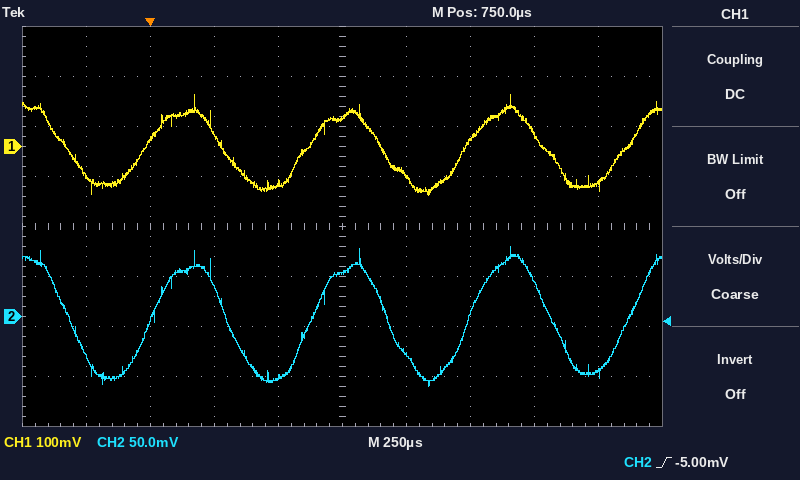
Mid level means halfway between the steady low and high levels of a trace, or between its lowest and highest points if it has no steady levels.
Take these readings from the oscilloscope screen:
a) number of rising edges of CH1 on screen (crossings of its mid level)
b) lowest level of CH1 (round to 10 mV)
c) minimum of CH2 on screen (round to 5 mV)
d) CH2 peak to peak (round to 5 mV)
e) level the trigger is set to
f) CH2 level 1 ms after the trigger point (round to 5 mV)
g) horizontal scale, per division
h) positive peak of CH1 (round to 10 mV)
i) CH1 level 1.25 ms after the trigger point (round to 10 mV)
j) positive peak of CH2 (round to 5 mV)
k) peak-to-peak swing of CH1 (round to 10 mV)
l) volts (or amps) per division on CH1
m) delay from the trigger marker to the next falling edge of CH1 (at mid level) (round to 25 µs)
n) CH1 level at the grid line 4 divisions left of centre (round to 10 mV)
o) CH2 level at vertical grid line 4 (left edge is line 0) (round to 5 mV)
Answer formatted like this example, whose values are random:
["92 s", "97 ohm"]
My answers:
["4", "-100 mV", "-70 mV", "140 mV", "-5.00 mV", "-35 mV", "250 µs", "100 mV", "10 mV", "70 mV", "200 mV", "100 mV", "275 µs", "-60 mV", "-60 mV"]
